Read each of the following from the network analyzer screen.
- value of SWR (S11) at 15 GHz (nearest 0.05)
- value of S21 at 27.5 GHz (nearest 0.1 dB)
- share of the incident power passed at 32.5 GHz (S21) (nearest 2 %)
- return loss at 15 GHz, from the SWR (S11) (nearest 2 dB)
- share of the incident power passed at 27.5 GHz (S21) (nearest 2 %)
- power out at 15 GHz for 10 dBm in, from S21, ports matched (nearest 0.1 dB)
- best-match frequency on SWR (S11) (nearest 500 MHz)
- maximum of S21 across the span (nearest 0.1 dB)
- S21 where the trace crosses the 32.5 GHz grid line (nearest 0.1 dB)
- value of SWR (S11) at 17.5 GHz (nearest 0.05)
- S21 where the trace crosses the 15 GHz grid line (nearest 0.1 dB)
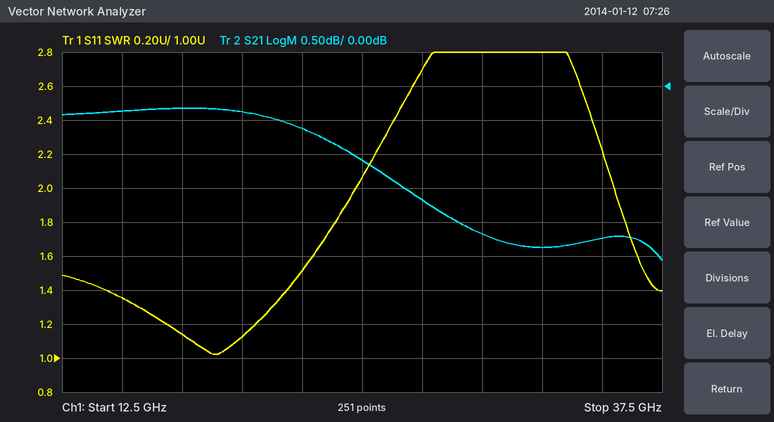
1.35
-1.7 dB
58 %
16 dB
68 %
9.6 dBm
19.0 GHz
-0.3 dB
-2.4 dB
1.15
-0.4 dB
